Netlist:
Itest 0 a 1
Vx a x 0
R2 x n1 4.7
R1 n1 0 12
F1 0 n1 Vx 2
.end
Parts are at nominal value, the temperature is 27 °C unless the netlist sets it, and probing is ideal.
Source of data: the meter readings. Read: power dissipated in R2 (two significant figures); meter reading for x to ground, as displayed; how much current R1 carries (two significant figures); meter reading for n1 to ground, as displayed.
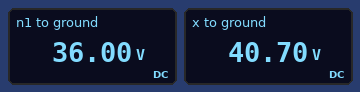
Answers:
4.7 W
40.70 V
3.0 A
36.00 V
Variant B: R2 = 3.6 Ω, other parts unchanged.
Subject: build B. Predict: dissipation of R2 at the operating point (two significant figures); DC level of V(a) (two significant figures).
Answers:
3.6 W
40 V
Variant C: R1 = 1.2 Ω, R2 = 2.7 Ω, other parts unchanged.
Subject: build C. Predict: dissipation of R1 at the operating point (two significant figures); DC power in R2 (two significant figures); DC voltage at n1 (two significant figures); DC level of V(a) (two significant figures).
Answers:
11 W
2.7 W
3.6 V
6.3 V
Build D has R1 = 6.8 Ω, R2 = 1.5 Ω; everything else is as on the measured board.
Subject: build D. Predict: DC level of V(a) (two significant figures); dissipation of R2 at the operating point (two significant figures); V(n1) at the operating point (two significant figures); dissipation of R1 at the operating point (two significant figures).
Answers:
22 V
1.5 W
20 V
61 W
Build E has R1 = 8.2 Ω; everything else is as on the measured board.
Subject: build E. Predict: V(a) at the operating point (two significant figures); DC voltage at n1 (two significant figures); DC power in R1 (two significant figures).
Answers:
29 V
25 V
74 W
